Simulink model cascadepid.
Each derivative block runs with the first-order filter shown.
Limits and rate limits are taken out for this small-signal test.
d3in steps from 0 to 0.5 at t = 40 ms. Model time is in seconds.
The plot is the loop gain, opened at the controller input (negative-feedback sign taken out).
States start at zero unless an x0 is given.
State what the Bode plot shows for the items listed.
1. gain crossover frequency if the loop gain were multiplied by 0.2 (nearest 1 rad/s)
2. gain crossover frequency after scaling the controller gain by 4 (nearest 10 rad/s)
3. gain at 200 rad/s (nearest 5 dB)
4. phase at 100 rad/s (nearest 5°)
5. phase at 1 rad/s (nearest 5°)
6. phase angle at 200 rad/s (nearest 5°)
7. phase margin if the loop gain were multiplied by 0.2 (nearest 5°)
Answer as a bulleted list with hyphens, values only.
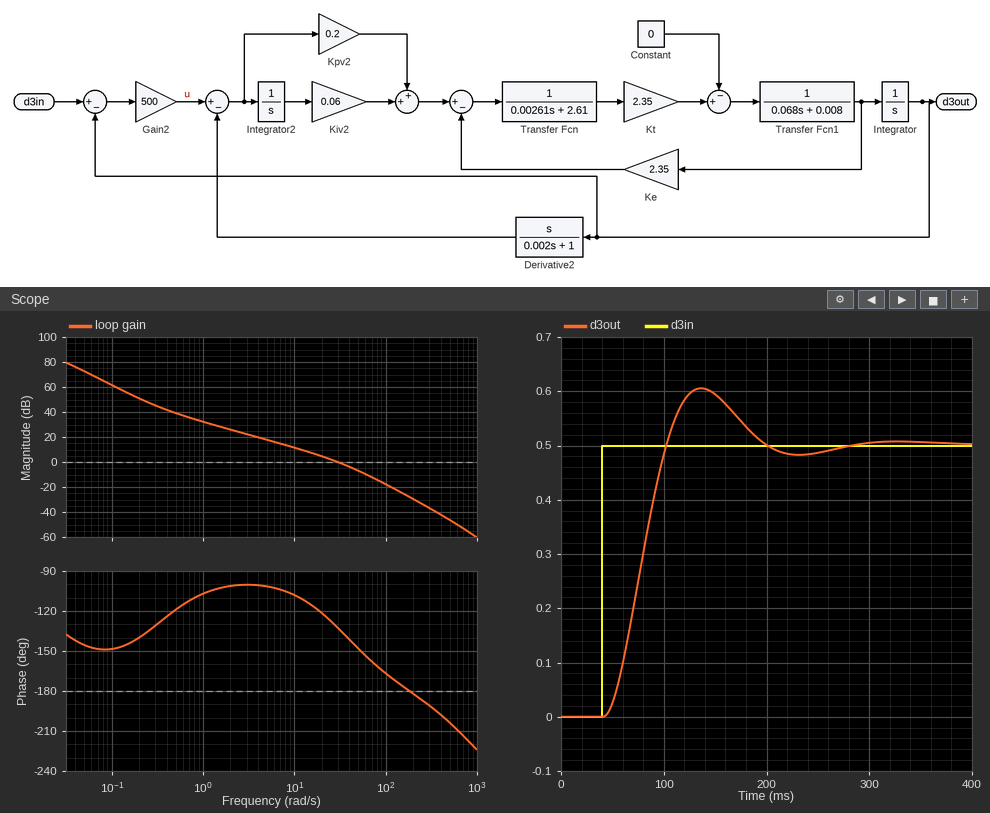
- 8 rad/s
- 70 rad/s
- -30 dB
- -165°
- -105°
- -180°
- 75°
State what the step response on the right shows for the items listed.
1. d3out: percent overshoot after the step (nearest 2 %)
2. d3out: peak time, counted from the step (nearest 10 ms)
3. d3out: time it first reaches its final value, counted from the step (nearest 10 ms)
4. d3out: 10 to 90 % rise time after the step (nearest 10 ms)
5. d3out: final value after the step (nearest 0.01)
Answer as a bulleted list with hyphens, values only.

- 20 %
- 100 ms
- 60 ms
- 40 ms
- 0.50
